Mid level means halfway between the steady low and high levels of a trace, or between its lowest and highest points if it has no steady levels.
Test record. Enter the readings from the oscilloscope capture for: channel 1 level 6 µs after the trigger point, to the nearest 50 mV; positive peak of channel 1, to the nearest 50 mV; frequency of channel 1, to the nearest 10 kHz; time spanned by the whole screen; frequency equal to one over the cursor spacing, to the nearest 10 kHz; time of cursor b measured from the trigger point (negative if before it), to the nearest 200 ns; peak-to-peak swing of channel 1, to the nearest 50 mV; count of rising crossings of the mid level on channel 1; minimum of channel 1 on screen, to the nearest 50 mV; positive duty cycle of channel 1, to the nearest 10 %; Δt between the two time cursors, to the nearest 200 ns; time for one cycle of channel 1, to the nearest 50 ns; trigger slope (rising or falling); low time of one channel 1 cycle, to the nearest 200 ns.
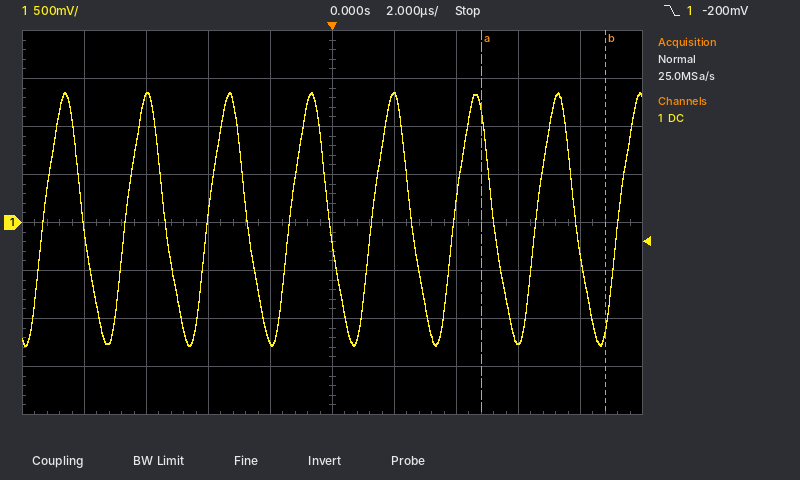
-1.25 V
1.35 V
380 kHz
20 µs
250 kHz
+8.8 µs
2.65 V
8
-1.30 V
50 %
4.0 µs
2.65 µs
falling
1.4 µs
